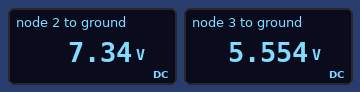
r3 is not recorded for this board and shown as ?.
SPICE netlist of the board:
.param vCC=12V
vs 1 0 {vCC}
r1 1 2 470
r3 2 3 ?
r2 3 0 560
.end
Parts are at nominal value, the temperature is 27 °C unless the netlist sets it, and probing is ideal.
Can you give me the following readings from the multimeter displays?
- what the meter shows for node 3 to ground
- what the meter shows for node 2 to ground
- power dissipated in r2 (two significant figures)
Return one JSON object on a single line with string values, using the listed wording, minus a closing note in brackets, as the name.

{"what the meter shows for node 3 to ground": "5.554 V", "what the meter shows for node 2 to ground": "7.34 V", "power dissipated in r2": "55 mW"}
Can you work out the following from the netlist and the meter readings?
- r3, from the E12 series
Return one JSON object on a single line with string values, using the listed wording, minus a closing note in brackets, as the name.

{"r3, from the E12 series": "180 Ω"}
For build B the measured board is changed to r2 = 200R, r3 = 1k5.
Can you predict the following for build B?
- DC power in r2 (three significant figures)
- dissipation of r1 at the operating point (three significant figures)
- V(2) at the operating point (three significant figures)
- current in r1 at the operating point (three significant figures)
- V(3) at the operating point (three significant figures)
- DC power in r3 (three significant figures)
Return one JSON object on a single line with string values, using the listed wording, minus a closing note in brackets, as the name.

{"DC power in r2": "6.12 mW", "dissipation of r1 at the operating point": "14.4 mW", "V(2) at the operating point": "9.40 V", "current in r1 at the operating point": "5.53 mA", "V(3) at the operating point": "1.11 V", "DC power in r3": "45.9 mW"}
